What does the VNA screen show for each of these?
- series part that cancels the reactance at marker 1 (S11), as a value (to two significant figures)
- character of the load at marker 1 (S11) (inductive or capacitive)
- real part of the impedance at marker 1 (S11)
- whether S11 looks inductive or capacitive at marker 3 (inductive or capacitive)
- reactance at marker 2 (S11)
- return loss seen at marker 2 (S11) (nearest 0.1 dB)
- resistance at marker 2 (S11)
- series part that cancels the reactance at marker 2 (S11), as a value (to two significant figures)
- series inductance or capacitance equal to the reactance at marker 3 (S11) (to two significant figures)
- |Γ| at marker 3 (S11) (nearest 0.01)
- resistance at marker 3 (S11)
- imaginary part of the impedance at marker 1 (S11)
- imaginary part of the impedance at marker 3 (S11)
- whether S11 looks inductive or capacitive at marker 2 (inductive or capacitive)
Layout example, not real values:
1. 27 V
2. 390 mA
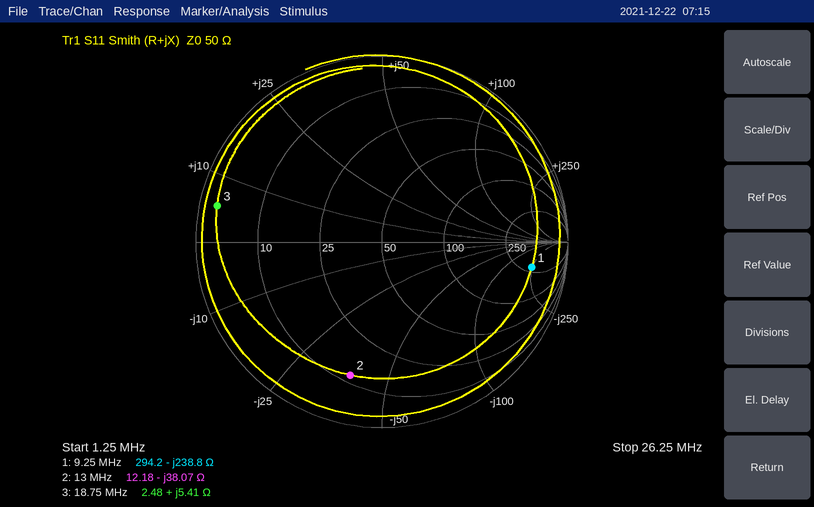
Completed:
1. 4.1 µH
2. capacitive
3. 294.2 Ω
4. inductive
5. -38.07 Ω
6. 2.7 dB
7. 12.18 Ω
8. 470 nH
9. 46 nH
10. 0.91
11. 2.48 Ω
12. -238.8 Ω
13. +5.41 Ω
14. capacitive
